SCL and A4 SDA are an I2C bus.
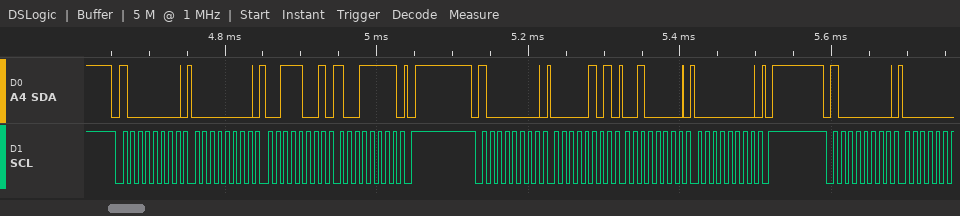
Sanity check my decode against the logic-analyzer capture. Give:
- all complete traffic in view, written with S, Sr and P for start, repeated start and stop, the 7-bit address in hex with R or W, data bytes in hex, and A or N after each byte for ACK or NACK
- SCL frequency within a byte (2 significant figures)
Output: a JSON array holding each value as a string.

["S 40W A 00 A 39 A 9F A P S 40W A 05 A 20 A 00 A P S 40W A", "100 kHz"]
